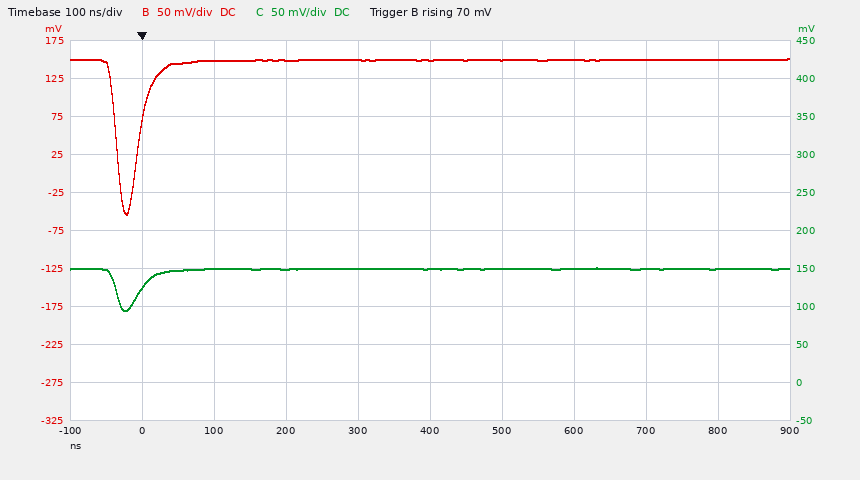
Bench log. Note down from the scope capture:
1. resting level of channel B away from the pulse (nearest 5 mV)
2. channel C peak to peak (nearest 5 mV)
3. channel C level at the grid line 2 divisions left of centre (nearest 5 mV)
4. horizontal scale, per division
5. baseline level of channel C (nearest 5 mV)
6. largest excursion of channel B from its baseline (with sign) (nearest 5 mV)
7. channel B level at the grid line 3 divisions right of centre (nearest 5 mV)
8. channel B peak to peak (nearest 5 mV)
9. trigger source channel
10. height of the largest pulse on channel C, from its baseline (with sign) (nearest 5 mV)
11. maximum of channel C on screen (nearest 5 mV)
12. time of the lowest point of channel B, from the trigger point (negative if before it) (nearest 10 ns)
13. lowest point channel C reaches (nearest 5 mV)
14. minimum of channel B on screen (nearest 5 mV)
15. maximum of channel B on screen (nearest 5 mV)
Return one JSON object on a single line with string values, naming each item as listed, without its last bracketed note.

{"resting level of channel B away from the pulse": "150 mV", "channel C peak to peak": "55 mV", "channel C level at the grid line 2 divisions left of centre": "150 mV", "horizontal scale, per division": "100 ns", "baseline level of channel C": "150 mV", "largest excursion of channel B from its baseline (with sign)": "-205 mV", "channel B level at the grid line 3 divisions right of centre": "150 mV", "channel B peak to peak": "205 mV", "trigger source channel": "channel B", "height of the largest pulse on channel C, from its baseline (with sign)": "-55 mV", "maximum of channel C on screen": "150 mV", "time of the lowest point of channel B, from the trigger point (negative if before it)": "-20 ns", "lowest point channel C reaches": "95 mV", "minimum of channel B on screen": "-55 mV", "maximum of channel B on screen": "150 mV"}
